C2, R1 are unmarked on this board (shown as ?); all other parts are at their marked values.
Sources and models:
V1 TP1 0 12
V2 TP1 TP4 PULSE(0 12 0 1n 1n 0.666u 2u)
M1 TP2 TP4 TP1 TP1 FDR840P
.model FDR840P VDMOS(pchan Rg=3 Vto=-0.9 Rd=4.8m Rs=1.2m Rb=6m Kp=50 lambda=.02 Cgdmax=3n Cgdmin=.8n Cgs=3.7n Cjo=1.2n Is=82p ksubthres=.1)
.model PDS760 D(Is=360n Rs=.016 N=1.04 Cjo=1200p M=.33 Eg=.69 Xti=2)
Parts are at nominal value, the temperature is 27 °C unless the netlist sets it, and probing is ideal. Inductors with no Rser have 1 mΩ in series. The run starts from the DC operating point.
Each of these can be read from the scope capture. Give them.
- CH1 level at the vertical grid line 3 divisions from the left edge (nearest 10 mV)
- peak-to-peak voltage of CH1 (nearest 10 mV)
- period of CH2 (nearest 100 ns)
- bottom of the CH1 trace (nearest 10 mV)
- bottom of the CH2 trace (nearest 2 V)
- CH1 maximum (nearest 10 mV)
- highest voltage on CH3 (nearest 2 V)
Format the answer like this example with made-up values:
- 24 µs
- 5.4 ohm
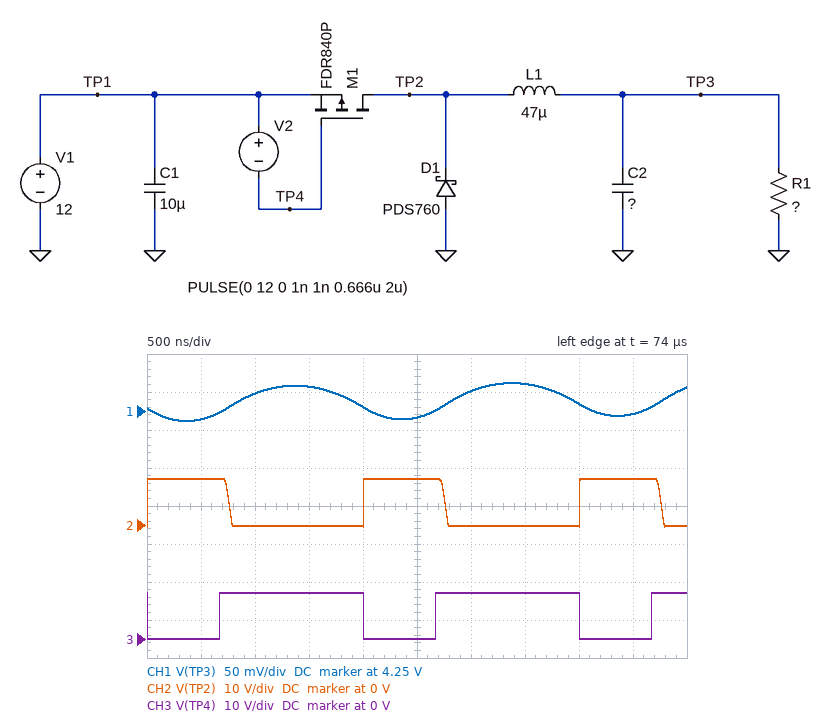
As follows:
- 4.28 V
- 50 mV
- 2.0 µs
- 4.24 V
- 0 V
- 4.29 V
- 12 V
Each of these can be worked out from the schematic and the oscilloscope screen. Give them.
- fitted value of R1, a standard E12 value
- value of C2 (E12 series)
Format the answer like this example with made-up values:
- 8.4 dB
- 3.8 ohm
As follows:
- 12 Ω
- 680 nF
